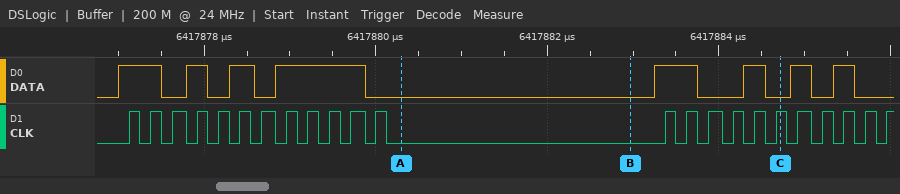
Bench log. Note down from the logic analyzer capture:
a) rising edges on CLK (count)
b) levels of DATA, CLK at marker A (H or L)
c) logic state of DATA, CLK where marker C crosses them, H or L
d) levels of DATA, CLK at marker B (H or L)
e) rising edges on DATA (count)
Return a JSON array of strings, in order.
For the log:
["23", "DATA=L, CLK=L", "DATA=L, CLK=H", "DATA=L, CLK=L", "8"]
